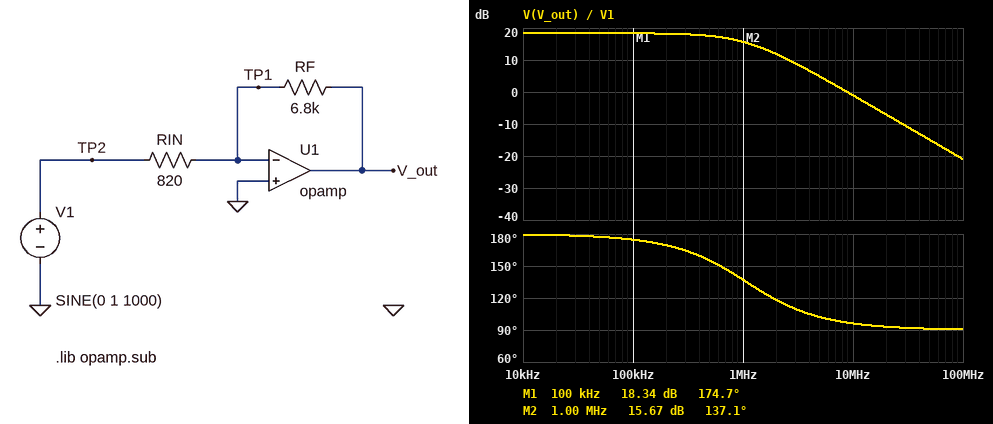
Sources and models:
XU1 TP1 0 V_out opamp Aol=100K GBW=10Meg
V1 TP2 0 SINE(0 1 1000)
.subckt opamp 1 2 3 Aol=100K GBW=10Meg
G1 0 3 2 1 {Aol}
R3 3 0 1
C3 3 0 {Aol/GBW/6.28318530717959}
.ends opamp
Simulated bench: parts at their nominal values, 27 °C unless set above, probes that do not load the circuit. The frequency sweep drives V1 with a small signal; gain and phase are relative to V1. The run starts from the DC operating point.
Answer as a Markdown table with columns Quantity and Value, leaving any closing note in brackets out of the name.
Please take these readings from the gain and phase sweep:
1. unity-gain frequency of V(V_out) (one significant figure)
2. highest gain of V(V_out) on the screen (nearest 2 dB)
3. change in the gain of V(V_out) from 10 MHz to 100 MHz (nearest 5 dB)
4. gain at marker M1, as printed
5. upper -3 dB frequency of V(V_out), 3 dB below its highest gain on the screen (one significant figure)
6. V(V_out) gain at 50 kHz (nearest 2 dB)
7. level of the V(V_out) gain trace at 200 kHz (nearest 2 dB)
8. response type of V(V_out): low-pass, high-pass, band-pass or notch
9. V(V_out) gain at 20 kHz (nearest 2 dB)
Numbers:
| Quantity | Value |
|---|---|
| unity-gain frequency of V(V_out) | 9 MHz |
| highest gain of V(V_out) on the screen | 18 dB |
| change in the gain of V(V_out) from 10 MHz to 100 MHz | -20 dB |
| gain at marker M1, as printed | 18.34 dB |
| upper -3 dB frequency of V(V_out), 3 dB below its highest gain on the screen | 1 MHz |
| V(V_out) gain at 50 kHz | 18 dB |
| level of the V(V_out) gain trace at 200 kHz | 18 dB |
| response type of V(V_out): low-pass, high-pass, band-pass or notch | low-pass |
| V(V_out) gain at 20 kHz | 18 dB |
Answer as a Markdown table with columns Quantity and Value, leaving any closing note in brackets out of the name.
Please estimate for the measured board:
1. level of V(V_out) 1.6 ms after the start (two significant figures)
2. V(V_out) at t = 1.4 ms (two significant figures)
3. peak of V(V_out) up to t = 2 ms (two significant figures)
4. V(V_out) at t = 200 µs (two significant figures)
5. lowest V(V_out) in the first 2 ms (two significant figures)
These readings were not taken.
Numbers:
| Quantity | Value |
|---|---|
| level of V(V_out) 1.6 ms after the start | 4.9 V |
| V(V_out) at t = 1.4 ms | -4.9 V |
| peak of V(V_out) up to t = 2 ms | 8.3 V |
| V(V_out) at t = 200 µs | -7.9 V |
| lowest V(V_out) in the first 2 ms | -8.3 V |
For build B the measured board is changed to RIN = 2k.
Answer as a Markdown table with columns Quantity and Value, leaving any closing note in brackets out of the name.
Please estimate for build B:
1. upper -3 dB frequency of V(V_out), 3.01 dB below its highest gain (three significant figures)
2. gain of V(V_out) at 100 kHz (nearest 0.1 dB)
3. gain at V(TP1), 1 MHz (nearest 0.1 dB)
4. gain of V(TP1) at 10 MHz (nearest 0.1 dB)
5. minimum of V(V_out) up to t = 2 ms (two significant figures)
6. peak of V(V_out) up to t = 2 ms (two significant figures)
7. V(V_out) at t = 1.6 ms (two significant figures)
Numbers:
| Quantity | Value |
|---|---|
| upper -3 dB frequency of V(V_out), 3.01 dB below its highest gain | 2.27 MHz |
| gain of V(V_out) at 100 kHz | 10.6 dB |
| gain at V(TP1), 1 MHz | -10.1 dB |
| gain of V(TP1) at 10 MHz | -2.5 dB |
| minimum of V(V_out) up to t = 2 ms | -3.4 V |
| peak of V(V_out) up to t = 2 ms | 3.4 V |
| V(V_out) at t = 1.6 ms | 2.0 V |
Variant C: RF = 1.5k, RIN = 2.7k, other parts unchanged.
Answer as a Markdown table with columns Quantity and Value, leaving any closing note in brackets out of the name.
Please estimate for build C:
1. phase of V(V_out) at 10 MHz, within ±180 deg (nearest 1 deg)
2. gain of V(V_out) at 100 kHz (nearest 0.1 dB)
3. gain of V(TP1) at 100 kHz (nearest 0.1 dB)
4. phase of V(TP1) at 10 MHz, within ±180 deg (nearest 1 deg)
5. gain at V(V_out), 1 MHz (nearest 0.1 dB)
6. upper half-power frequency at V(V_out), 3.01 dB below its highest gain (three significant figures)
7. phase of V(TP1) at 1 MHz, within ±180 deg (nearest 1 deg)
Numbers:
| Quantity | Value |
|---|---|
| phase of V(V_out) at 10 MHz, within ±180 deg | 123 deg |
| gain of V(V_out) at 100 kHz | -5.1 dB |
| gain of V(TP1) at 100 kHz | -45.1 dB |
| phase of V(TP1) at 10 MHz, within ±180 deg | 33 deg |
| gain at V(V_out), 1 MHz | -5.2 dB |
| upper half-power frequency at V(V_out), 3.01 dB below its highest gain | 6.43 MHz |
| phase of V(TP1) at 1 MHz, within ±180 deg | 81 deg |
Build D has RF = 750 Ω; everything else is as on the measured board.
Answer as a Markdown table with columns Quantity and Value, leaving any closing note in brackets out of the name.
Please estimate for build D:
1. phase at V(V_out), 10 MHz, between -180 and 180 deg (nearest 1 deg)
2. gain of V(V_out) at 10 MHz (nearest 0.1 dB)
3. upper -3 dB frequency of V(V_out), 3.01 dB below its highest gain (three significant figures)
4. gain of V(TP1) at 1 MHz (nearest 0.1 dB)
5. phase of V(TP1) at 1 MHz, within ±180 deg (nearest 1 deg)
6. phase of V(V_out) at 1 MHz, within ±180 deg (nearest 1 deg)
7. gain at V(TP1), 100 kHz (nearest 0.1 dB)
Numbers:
| Quantity | Value |
|---|---|
| phase at V(V_out), 10 MHz, between -180 and 180 deg | 118 deg |
| gain of V(V_out) at 10 MHz | -7.5 dB |
| upper -3 dB frequency of V(V_out), 3.01 dB below its highest gain | 5.22 MHz |
| gain of V(TP1) at 1 MHz | -20.9 dB |
| phase of V(TP1) at 1 MHz, within ±180 deg | 79 deg |
| phase of V(V_out) at 1 MHz, within ±180 deg | 169 deg |
| gain at V(TP1), 100 kHz | -40.8 dB |
